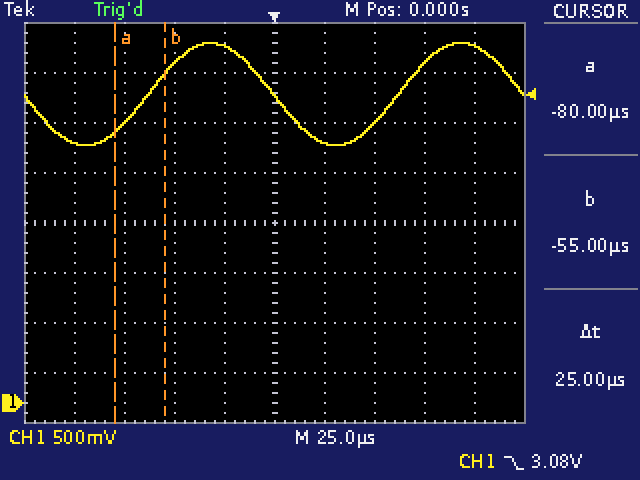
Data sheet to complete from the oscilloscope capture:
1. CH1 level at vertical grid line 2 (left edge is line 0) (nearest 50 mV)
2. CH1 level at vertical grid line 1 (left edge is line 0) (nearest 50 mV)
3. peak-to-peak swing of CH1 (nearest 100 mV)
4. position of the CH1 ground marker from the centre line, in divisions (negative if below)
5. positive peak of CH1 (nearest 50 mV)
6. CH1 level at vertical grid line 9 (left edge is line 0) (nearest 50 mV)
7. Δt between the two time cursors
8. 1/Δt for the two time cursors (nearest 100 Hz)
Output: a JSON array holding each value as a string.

["2.80 V", "2.60 V", "1.00 V", "-3.6 div", "3.60 V", "3.55 V", "25 µs", "40.0 kHz"]
